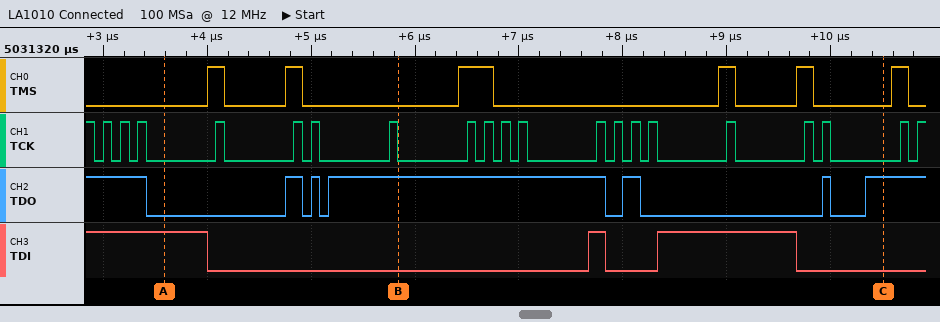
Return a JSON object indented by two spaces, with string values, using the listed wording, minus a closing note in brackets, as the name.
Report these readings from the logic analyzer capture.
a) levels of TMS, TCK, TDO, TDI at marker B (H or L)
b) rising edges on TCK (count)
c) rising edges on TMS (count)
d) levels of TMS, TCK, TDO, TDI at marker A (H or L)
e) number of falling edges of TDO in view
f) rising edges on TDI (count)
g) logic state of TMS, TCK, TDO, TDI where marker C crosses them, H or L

{
  "levels of TMS, TCK, TDO, TDI at marker B": "TMS=L, TCK=L, TDO=H, TDI=L",
  "rising edges on TCK": "20",
  "rising edges on TMS": "6",
  "levels of TMS, TCK, TDO, TDI at marker A": "TMS=L, TCK=L, TDO=L, TDI=H",
  "number of falling edges of TDO in view": "6",
  "rising edges on TDI": "2",
  "logic state of TMS, TCK, TDO, TDI where marker C crosses them, H or L": "TMS=L, TCK=L, TDO=H, TDI=L"
}
